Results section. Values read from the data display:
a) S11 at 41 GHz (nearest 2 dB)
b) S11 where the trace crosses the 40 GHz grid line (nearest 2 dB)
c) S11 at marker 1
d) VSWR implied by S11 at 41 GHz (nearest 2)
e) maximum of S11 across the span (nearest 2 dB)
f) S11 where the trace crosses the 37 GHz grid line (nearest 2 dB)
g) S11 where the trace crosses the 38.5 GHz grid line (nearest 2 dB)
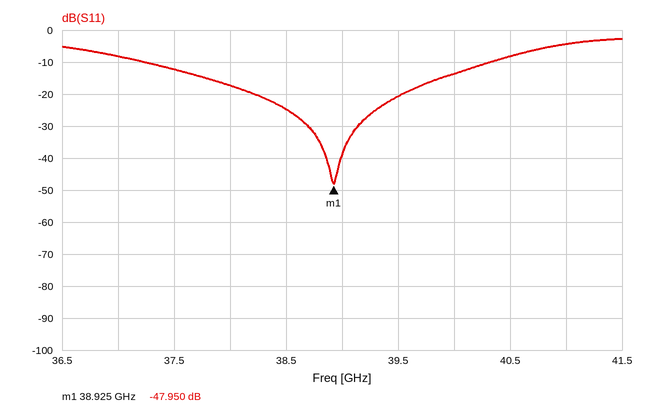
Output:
-4 dB
-14 dB
-47.950 dB
4
-2 dB
-8 dB
-24 dB
